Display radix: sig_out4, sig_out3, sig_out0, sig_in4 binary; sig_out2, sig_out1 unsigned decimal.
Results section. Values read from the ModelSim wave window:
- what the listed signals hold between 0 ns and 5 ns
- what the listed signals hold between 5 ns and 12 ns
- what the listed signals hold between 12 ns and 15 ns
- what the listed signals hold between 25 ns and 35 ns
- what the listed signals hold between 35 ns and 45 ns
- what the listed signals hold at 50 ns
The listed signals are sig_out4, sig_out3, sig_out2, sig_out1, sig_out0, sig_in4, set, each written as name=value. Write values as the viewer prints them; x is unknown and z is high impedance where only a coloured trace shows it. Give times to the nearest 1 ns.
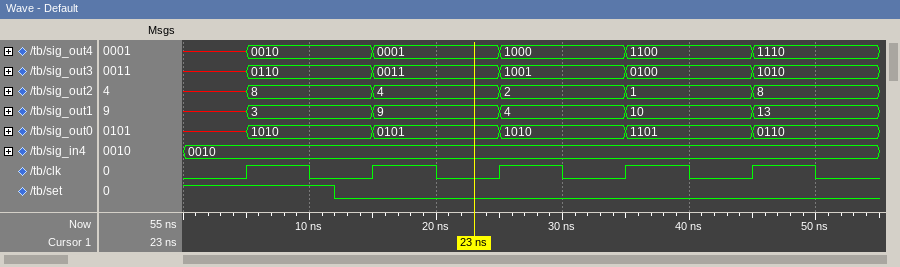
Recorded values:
sig_out4=x, sig_out3=x, sig_out2=x, sig_out1=x, sig_out0=x, sig_in4=0010, set=1
sig_out4=0010, sig_out3=0110, sig_out2=8, sig_out1=3, sig_out0=1010, sig_in4=0010, set=1
sig_out4=0010, sig_out3=0110, sig_out2=8, sig_out1=3, sig_out0=1010, sig_in4=0010, set=0
sig_out4=1000, sig_out3=1001, sig_out2=2, sig_out1=4, sig_out0=1010, sig_in4=0010, set=0
sig_out4=1100, sig_out3=0100, sig_out2=1, sig_out1=10, sig_out0=1101, sig_in4=0010, set=0
sig_out4=1110, sig_out3=1010, sig_out2=8, sig_out1=13, sig_out0=0110, sig_in4=0010, set=0
